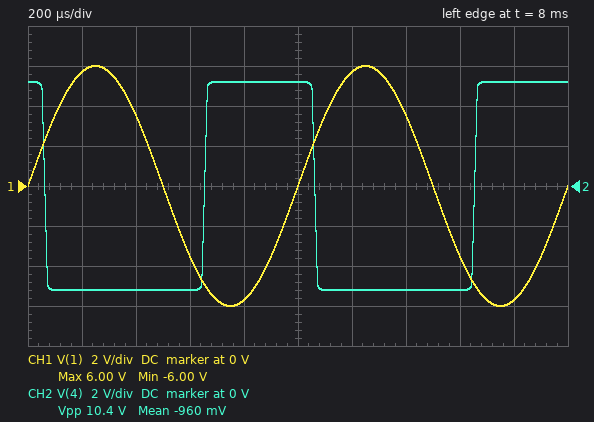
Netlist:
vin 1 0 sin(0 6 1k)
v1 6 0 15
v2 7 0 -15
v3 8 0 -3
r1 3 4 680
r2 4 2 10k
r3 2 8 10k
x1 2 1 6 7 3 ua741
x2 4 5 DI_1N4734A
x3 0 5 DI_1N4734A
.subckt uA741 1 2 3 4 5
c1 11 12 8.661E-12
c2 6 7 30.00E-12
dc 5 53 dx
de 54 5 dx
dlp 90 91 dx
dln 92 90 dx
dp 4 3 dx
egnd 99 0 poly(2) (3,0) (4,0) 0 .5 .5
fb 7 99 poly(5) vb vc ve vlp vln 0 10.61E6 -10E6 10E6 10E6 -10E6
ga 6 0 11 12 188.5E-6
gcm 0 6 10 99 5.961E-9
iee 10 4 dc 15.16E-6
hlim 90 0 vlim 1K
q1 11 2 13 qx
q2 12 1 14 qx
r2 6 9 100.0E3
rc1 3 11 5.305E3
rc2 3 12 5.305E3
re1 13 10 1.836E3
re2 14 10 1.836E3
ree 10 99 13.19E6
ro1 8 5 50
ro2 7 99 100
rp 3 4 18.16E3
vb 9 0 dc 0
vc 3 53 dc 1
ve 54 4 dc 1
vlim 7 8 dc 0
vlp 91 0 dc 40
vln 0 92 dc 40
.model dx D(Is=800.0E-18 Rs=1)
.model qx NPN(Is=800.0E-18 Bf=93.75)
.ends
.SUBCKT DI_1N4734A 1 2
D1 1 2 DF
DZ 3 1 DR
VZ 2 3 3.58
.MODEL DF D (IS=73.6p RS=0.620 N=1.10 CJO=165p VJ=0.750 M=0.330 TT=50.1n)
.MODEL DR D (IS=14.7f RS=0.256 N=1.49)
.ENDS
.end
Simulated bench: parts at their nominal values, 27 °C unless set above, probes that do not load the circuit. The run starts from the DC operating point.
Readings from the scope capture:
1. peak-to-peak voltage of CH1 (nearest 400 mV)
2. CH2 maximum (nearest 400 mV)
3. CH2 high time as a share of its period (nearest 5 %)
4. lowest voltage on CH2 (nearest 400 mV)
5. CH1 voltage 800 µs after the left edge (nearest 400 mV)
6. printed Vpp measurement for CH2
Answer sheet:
12.0 V
5.2 V
40 %
-5.2 V
-5.6 V
10.4 V
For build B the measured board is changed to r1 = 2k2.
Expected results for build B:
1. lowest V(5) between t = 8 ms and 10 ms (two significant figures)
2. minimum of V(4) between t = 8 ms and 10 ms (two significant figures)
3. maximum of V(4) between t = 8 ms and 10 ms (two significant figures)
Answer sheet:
-510 mV
-5.1 V
5.1 V
